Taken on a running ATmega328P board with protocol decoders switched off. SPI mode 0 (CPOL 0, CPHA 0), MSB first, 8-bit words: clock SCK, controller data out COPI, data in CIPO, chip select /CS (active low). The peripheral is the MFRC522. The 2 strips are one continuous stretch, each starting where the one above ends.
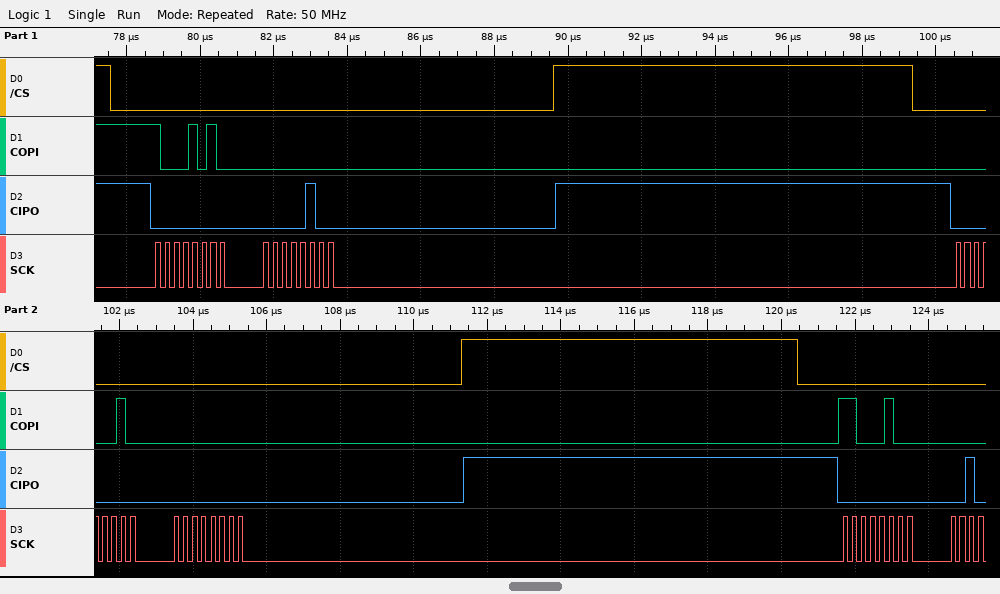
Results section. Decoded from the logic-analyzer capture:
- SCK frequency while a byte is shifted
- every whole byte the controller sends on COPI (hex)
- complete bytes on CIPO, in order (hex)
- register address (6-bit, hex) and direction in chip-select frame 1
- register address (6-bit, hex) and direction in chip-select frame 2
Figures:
4 MHz
0x8A 0x00 0x02 0x00 0xC4
0x00 0x04 0x00 0x00 0x00
0x05 read
0x01 write
